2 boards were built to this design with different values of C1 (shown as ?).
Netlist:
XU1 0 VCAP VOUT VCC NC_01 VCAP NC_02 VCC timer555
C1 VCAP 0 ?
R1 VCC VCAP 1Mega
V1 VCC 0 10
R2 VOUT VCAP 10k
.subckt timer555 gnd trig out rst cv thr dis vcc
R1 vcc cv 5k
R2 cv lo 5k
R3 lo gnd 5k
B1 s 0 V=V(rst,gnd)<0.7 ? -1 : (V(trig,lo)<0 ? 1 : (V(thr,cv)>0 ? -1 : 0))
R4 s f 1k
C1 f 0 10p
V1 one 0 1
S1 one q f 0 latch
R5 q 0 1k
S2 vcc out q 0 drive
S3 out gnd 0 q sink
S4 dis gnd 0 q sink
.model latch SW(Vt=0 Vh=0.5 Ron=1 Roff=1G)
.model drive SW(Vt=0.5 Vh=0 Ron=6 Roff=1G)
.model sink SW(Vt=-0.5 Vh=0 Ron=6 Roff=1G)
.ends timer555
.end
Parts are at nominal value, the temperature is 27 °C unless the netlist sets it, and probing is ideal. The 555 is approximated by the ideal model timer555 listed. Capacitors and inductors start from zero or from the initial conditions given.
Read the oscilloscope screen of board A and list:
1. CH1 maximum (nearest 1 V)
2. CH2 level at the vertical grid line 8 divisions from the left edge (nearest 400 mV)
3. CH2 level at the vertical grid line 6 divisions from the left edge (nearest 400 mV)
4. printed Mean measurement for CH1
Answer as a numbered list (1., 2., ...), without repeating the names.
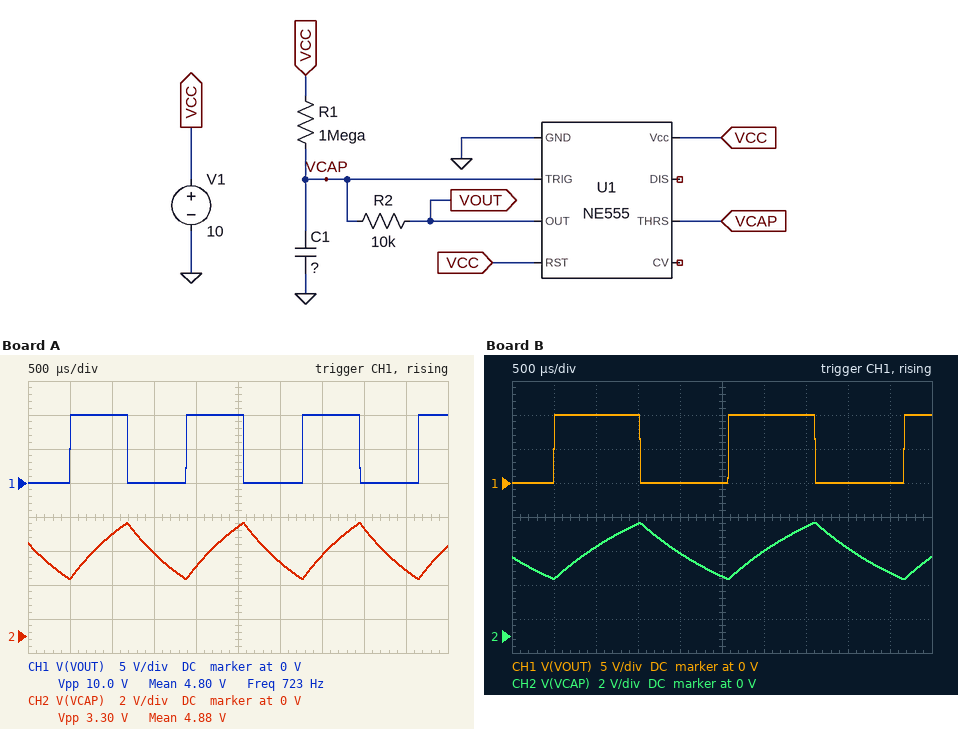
1. 10 V
2. 6.4 V
3. 4.4 V
4. 4.80 V
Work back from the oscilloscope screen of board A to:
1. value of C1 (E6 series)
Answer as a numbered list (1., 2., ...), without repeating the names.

1. 100 nF
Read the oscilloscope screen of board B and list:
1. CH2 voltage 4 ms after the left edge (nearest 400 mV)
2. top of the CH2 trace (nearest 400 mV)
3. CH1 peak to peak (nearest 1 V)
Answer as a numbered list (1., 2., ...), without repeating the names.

1. 5.2 V
2. 6.8 V
3. 10 V
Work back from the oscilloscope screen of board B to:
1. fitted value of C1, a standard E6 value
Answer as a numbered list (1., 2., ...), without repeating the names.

1. 150 nF
